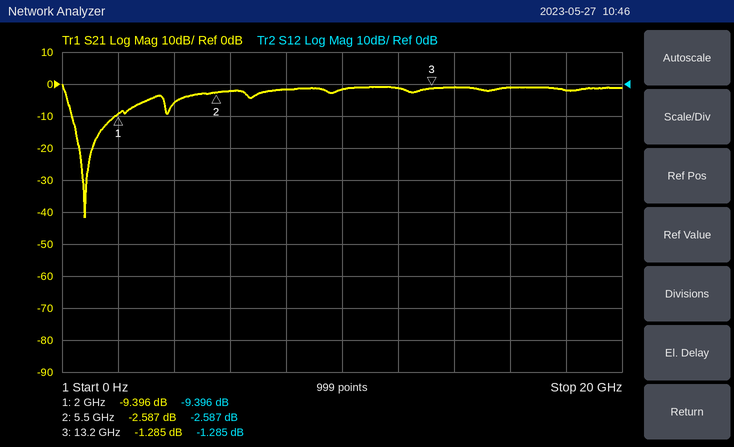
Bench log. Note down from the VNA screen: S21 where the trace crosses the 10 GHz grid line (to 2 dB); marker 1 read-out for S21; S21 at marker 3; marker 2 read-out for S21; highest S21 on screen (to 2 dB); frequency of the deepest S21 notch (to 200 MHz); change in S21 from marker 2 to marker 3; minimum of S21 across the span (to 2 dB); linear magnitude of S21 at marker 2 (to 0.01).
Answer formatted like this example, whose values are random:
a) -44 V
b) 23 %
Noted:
a) -2 dB
b) -9.396 dB
c) -1.285 dB
d) -2.587 dB
e) 0 dB
f) 800 MHz
g) 1.302 dB
h) -42 dB
i) 0.74
